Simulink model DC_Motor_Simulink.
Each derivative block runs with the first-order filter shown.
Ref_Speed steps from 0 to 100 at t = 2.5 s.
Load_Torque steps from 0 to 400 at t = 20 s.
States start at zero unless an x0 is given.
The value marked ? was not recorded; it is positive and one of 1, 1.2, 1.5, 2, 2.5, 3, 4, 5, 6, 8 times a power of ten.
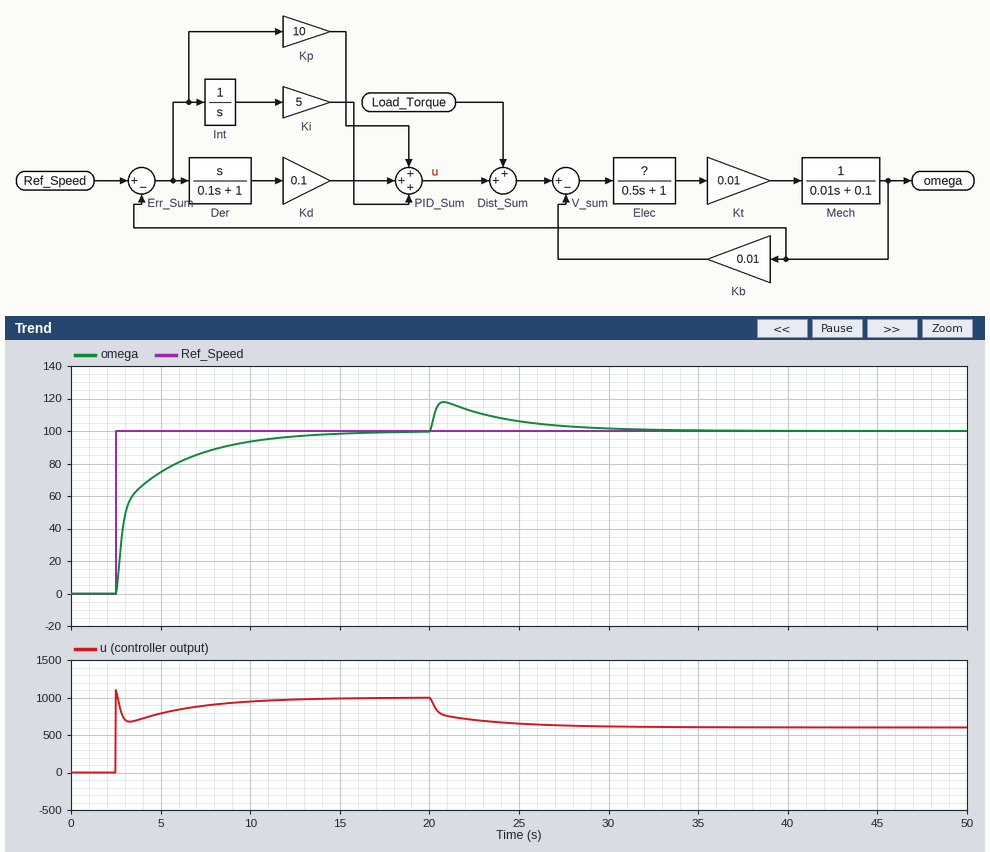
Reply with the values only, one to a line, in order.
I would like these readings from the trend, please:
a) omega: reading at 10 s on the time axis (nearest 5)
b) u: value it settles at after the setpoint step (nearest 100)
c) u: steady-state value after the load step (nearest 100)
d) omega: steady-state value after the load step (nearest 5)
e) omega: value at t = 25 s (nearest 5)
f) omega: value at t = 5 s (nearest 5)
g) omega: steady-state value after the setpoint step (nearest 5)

95
1000
600
100
105
75
100
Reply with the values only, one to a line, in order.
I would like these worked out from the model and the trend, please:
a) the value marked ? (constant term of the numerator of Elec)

1
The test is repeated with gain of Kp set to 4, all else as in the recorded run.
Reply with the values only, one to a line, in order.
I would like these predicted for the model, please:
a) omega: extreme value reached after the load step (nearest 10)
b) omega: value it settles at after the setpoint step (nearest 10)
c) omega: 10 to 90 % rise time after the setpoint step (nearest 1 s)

120
100
5 s
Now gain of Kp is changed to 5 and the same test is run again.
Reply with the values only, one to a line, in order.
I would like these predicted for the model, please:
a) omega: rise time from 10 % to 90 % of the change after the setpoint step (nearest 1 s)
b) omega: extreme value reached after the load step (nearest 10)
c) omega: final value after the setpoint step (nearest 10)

5 s
120
100
